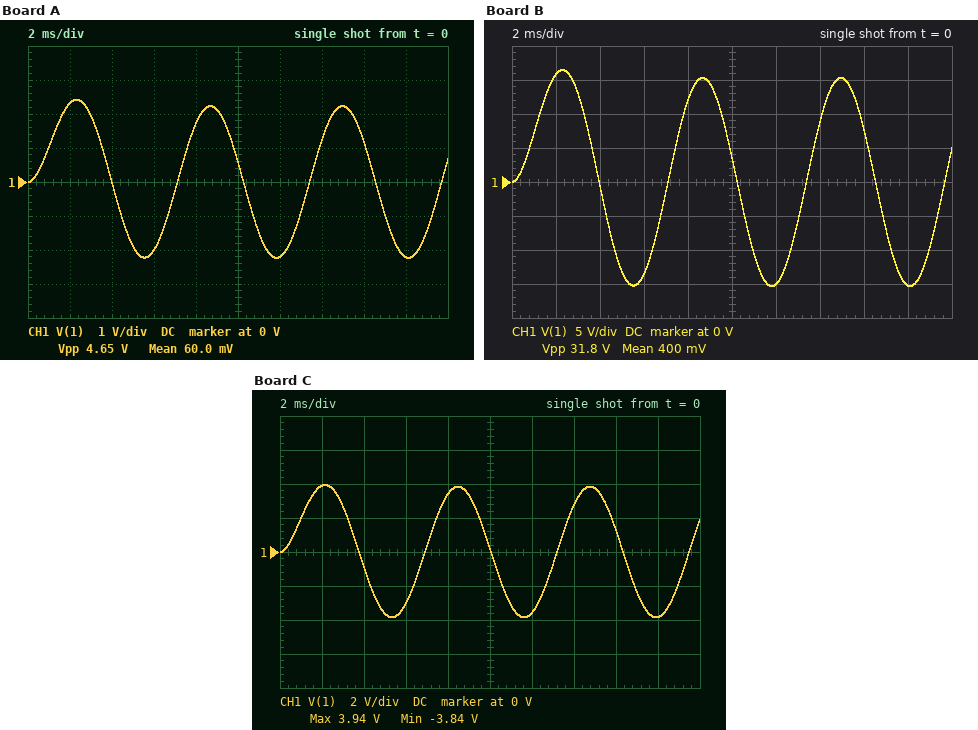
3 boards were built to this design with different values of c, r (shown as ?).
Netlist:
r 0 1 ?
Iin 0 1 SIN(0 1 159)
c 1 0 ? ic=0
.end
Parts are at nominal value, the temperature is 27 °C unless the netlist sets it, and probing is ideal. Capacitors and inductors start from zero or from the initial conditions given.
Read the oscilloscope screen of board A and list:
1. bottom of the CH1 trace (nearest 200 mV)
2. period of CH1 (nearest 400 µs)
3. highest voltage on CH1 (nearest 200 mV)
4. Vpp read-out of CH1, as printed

-2.2 V
6.4 ms
2.4 V
4.65 V
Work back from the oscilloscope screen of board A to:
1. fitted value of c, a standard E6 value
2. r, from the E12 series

330 µF
3.3 Ω
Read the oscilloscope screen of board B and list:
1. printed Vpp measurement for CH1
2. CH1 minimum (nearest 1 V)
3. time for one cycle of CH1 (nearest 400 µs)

31.8 V
-15 V
6.4 ms
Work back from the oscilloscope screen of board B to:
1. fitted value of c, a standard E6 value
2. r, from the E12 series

47 µF
22 Ω
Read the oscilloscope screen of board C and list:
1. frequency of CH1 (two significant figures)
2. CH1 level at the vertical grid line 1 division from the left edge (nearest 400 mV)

160 Hz
4.0 V
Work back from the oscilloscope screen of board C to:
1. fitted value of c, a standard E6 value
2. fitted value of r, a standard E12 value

150 µF
4.7 Ω
